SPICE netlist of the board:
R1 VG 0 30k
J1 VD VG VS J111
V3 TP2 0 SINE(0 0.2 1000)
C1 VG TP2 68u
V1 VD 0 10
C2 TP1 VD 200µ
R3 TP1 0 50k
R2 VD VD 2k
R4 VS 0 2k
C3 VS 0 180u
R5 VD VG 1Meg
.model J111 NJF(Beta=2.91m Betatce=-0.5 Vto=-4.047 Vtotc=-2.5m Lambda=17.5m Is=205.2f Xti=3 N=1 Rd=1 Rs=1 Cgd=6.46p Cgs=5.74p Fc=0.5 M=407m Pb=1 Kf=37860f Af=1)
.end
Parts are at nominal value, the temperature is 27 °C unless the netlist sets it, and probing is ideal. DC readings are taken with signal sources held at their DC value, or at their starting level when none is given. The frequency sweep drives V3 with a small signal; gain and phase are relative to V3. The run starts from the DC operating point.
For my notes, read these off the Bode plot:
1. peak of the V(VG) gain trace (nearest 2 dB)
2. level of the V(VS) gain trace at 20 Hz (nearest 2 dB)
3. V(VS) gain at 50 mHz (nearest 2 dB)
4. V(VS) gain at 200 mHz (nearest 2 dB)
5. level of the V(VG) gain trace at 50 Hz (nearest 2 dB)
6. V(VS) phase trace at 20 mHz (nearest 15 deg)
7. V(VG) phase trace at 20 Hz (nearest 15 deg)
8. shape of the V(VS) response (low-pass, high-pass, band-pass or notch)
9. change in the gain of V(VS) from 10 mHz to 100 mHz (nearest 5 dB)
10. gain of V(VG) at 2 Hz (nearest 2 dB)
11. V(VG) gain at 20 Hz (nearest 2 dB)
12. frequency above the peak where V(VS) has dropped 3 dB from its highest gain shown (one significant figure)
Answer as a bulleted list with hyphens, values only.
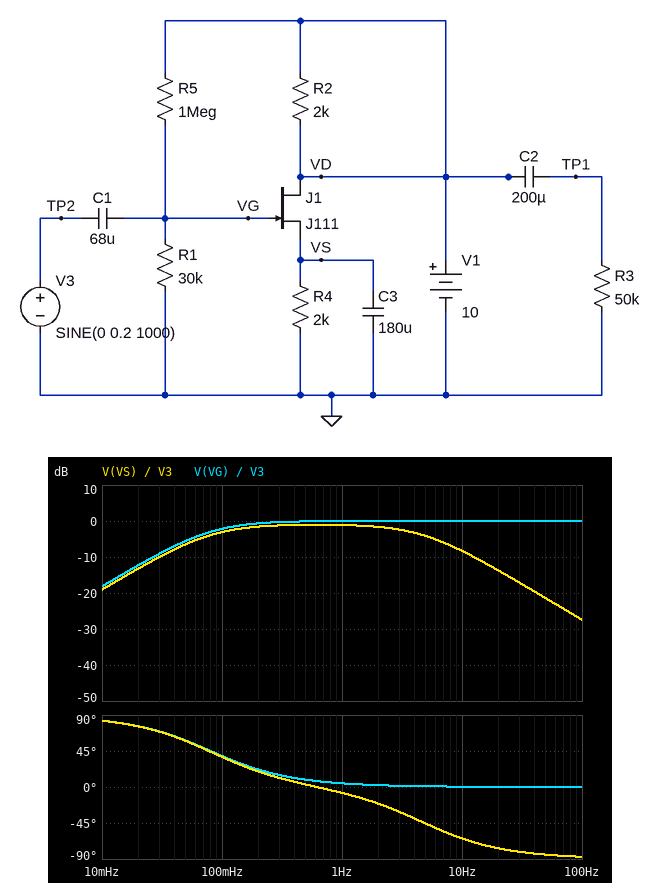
- 0 dB
- -14 dB
- -6 dB
- -2 dB
- 0 dB
- 75 deg
- 0 deg
- band-pass
- 15 dB
- 0 dB
- 0 dB
- 5 Hz
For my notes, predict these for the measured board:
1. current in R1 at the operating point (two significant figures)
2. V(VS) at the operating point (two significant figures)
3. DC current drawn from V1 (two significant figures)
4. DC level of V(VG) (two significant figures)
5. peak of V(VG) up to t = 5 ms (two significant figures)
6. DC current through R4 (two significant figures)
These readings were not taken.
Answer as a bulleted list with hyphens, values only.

- 9.7 µA
- 3.6 V
- 1.8 mA
- 290 mV
- 490 mV
- 1.8 mA
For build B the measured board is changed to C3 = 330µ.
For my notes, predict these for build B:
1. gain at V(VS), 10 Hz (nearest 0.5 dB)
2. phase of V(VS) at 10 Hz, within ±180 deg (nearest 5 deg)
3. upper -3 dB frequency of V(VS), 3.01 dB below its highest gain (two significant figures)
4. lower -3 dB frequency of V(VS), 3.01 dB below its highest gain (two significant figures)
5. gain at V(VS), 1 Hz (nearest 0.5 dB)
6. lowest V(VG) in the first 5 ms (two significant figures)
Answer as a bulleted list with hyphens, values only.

- -13.0 dB
- -75 deg
- 2.7 Hz
- 76 mHz
- -1.5 dB
- 91 mV
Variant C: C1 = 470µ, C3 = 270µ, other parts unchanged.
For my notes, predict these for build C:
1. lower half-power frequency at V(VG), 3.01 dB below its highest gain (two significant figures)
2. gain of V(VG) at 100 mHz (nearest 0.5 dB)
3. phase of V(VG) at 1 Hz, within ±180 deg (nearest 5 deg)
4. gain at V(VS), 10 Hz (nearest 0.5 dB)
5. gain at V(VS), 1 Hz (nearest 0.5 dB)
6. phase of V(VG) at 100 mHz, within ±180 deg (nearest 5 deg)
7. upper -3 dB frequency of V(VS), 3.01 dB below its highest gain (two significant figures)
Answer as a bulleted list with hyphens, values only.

- 12 mHz
- 0 dB
- 0 deg
- -11.5 dB
- -1.5 dB
- 5 deg
- 3.2 Hz
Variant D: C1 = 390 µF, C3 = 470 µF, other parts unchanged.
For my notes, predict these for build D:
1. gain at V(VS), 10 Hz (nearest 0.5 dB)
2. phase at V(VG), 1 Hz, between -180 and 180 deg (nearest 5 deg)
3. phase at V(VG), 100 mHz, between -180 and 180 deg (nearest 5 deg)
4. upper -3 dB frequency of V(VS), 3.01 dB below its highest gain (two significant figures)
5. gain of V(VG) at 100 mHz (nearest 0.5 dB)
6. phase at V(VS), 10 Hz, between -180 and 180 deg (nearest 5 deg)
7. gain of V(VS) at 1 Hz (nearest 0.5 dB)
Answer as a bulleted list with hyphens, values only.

- -16.0 dB
- 0 deg
- 10 deg
- 1.8 Hz
- 0 dB
- -80 deg
- -2.0 dB
